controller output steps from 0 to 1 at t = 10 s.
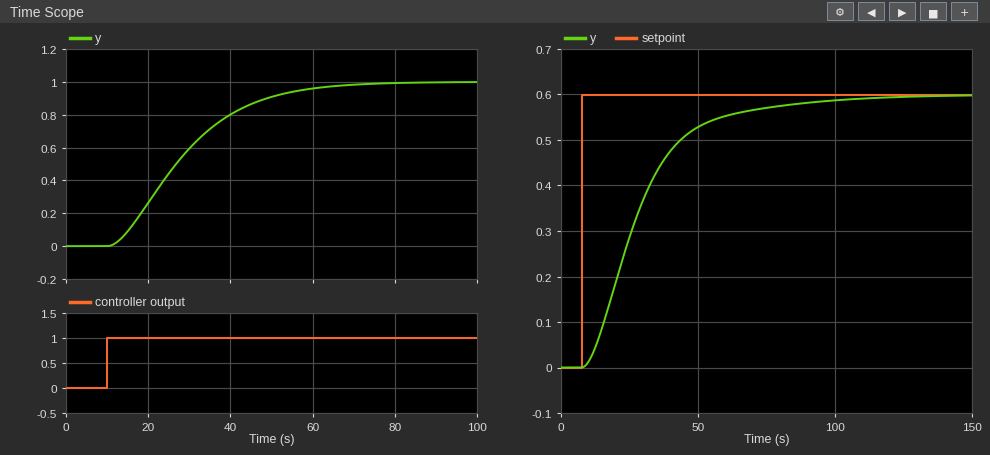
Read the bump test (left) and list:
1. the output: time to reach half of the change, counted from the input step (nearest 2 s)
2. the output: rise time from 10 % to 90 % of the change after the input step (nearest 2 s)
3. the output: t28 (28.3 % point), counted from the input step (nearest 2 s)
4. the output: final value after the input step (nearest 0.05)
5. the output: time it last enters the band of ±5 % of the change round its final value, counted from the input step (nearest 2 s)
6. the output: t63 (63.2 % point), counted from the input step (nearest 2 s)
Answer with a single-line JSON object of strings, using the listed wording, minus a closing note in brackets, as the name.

{"the output: time to reach half of the change, counted from the input step": "16 s", "the output: rise time from 10 % to 90 % of the change after the input step": "34 s", "the output: t28 (28.3 % point), counted from the input step": "10 s", "the output: final value after the input step": "1.00", "the output: time it last enters the band of ±5 % of the change round its final value, counted from the input step": "48 s", "the output: t63 (63.2 % point), counted from the input step": "22 s"}
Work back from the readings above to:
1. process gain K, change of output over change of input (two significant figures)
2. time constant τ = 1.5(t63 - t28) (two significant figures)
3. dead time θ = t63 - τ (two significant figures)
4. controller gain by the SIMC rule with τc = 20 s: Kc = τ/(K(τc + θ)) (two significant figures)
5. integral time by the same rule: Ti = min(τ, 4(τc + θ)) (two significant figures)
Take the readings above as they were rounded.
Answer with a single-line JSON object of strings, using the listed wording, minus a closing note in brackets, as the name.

{"process gain K, change of output over change of input": "1.0", "time constant τ = 1.5(t63 - t28)": "18 s", "dead time θ = t63 - τ": "4.0 s", "controller gain by the SIMC rule with τc = 20 s: Kc = τ/(K(τc + θ))": "0.75", "integral time by the same rule: Ti = min(τ, 4(τc + θ))": "18 s"}
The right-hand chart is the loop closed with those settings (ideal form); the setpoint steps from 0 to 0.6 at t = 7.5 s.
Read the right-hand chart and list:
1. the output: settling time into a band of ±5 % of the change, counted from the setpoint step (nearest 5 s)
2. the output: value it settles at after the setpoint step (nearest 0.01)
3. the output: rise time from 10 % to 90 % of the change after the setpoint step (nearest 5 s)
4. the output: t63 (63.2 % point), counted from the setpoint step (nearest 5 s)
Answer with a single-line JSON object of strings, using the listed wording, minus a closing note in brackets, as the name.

{"the output: settling time into a band of ±5 % of the change, counted from the setpoint step": "65 s", "the output: value it settles at after the setpoint step": "0.60", "the output: rise time from 10 % to 90 % of the change after the setpoint step": "40 s", "the output: t63 (63.2 % point), counted from the setpoint step": "25 s"}
